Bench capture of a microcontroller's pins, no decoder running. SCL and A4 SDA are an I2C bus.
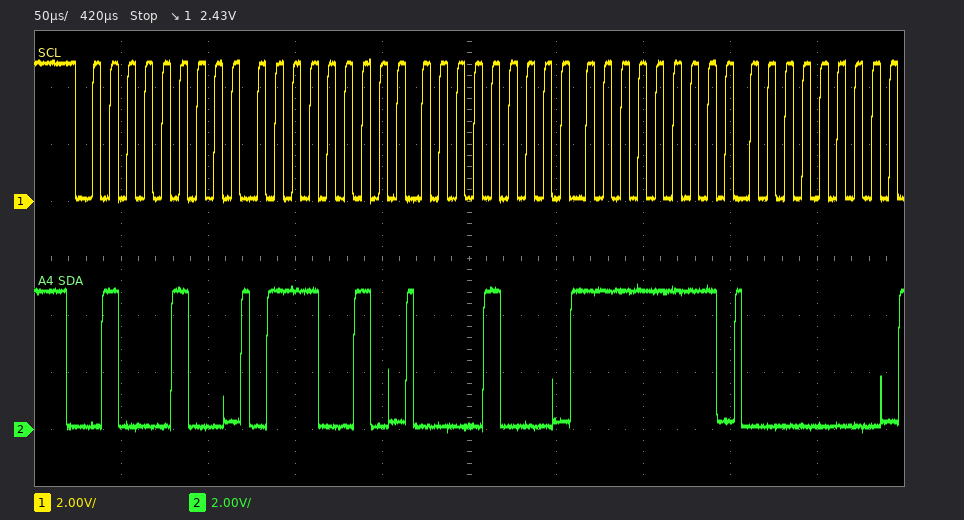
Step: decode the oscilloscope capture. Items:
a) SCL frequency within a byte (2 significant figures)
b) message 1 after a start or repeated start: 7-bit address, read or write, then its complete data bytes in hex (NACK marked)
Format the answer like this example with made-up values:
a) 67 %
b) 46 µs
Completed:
a) 100 kHz
b) 0x22 write: 72 08 FF 00
